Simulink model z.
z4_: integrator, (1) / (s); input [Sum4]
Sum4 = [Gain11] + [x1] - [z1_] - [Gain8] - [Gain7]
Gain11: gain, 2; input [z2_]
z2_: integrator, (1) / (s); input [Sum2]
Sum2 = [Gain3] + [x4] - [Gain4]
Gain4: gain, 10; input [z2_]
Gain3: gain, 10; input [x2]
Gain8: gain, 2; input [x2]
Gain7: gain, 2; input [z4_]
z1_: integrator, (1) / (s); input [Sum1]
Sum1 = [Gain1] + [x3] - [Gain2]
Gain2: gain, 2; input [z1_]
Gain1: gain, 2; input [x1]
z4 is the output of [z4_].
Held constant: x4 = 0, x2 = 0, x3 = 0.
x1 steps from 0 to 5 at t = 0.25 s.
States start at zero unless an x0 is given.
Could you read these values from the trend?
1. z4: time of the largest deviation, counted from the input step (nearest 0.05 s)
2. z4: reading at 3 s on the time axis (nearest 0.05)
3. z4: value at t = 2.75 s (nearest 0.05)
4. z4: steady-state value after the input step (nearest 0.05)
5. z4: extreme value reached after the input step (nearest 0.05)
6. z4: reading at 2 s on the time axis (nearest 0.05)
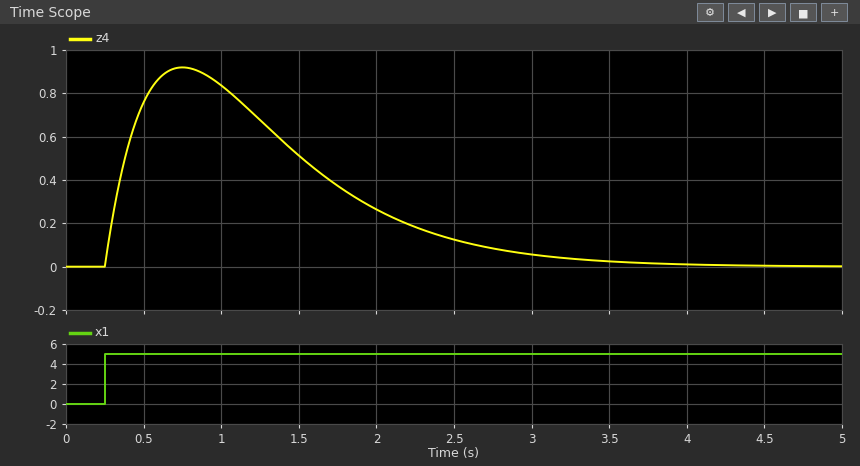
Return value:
0.50 s
0.05
0.10
0.00
0.90
0.25
